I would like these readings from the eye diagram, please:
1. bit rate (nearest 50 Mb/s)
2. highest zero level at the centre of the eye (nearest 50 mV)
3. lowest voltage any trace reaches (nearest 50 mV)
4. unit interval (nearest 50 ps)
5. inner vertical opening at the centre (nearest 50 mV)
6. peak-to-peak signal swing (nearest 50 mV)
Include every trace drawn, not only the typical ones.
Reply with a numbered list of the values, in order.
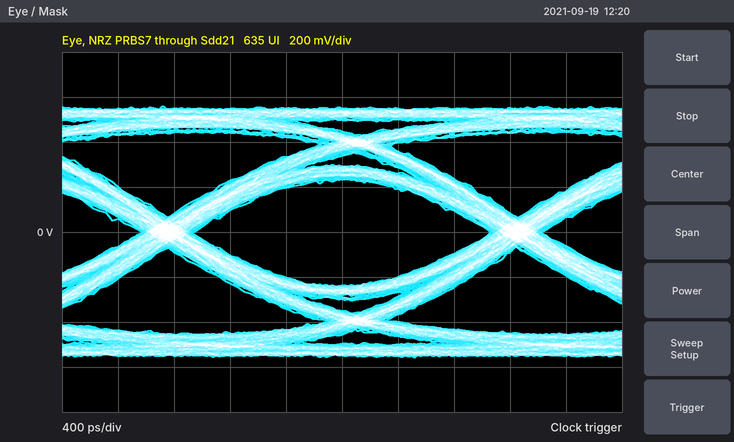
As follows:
1. 400 Mb/s
2. -250 mV
3. -550 mV
4. 2.50 ns
5. 450 mV
6. 1.10 V
